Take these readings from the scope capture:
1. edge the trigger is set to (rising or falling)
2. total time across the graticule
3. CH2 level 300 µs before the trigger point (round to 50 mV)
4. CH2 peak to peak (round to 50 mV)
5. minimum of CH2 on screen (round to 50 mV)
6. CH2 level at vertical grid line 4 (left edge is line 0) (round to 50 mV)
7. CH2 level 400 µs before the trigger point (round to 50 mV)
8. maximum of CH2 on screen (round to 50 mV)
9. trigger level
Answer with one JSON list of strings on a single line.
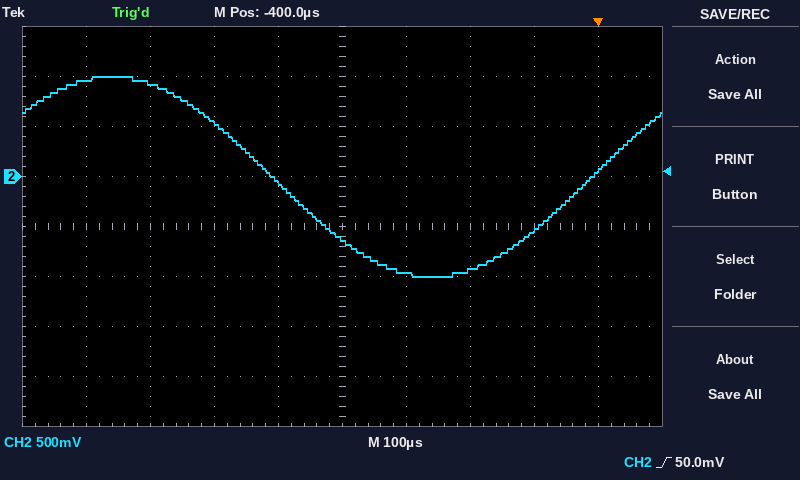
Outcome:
["rising", "1 ms", "-950 mV", "2.00 V", "-1.00 V", "-50 mV", "-600 mV", "1.00 V", "50.0 mV"]
